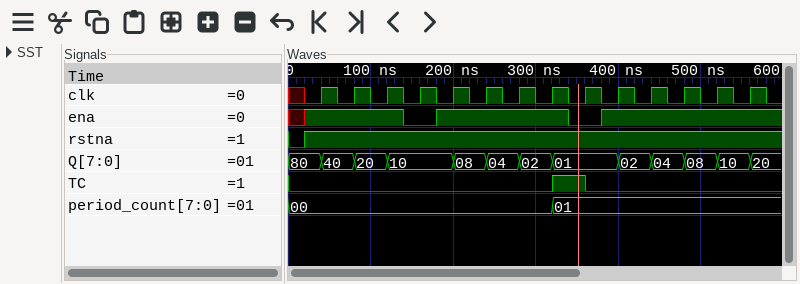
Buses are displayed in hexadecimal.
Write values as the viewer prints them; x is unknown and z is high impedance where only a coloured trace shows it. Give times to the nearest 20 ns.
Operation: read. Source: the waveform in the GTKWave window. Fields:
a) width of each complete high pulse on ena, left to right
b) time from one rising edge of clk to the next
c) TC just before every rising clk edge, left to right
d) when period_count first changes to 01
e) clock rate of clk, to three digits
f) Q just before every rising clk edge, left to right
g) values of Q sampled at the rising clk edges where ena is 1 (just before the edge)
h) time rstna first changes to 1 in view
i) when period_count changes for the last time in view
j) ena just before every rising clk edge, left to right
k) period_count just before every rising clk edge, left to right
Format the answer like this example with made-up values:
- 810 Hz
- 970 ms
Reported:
- 160 ns
- 40 ns
- 0 0 0 0 0 0 0 0 1 0 0 0 0 0
- 320 ns
- 25.0 MHz
- 80, 40, 20, 10, 10, 08, 04, 02, 01, 01, 02, 04, 08, 10
- 80, 40, 20, 10, 08, 04, 02, 01, 02, 04, 08, 10
- 20 ns
- 320 ns
- 1 1 1 0 1 1 1 1 0 1 1 1 1 1
- 00, 00, 00, 00, 00, 00, 00, 00, 01, 01, 01, 01, 01, 01
